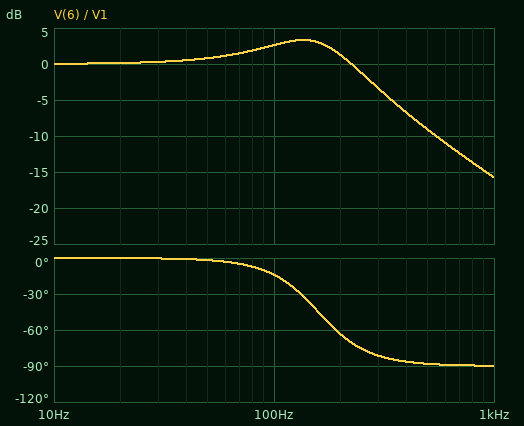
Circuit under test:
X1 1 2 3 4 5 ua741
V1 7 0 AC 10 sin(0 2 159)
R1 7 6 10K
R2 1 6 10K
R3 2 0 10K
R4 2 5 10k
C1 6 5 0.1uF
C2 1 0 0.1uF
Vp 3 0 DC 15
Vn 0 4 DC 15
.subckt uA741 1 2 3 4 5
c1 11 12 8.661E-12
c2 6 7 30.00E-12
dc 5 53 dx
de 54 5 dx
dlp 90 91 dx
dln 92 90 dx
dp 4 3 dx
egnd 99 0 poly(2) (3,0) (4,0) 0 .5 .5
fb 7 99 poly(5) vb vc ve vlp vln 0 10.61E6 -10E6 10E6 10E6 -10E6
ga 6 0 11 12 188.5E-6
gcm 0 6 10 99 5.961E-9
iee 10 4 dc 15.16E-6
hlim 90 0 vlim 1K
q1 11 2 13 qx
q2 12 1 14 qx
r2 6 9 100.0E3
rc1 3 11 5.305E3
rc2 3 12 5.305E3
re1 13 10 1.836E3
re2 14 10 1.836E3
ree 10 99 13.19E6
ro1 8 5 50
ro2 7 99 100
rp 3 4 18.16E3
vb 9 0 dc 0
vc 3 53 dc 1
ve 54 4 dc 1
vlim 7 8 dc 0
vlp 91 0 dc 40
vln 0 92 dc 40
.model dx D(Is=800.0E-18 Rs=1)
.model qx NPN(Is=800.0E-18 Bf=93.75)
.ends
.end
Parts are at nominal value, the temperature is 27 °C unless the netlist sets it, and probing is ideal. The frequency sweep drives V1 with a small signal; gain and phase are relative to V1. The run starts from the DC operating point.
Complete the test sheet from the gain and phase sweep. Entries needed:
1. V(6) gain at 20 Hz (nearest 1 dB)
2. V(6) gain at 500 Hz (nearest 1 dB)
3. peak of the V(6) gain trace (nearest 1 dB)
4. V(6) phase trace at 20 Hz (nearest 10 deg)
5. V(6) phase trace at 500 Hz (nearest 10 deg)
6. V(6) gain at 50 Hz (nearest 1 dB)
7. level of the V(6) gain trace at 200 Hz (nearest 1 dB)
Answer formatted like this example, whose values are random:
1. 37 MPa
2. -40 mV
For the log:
1. 0 dB
2. -9 dB
3. 3 dB
4. 0 deg
5. -90 deg
6. 1 dB
7. 1 dB
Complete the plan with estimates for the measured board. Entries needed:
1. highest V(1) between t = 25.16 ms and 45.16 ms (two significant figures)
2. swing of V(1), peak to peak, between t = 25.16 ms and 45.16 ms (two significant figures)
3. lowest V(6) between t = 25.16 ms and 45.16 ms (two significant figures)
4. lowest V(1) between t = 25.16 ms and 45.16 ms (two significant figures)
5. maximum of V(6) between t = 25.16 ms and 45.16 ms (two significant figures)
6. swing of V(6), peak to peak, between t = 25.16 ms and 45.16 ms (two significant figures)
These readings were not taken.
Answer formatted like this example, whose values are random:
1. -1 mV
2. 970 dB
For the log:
1. 2.0 V
2. 4.0 V
3. -2.8 V
4. -2.0 V
5. 2.8 V
6. 5.7 V
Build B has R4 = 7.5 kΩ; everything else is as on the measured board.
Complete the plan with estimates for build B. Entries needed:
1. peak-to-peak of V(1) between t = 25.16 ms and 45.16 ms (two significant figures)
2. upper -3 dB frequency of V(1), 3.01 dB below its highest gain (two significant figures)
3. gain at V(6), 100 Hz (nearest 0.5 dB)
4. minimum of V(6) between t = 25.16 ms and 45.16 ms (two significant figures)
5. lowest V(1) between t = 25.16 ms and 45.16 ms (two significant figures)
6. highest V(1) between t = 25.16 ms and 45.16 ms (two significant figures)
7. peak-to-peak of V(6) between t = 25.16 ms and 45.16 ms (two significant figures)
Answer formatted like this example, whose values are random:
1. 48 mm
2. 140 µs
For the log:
1. 3.2 V
2. 170 Hz
3. 1.5 dB
4. -2.3 V
5. -1.6 V
6. 1.6 V
7. 4.5 V
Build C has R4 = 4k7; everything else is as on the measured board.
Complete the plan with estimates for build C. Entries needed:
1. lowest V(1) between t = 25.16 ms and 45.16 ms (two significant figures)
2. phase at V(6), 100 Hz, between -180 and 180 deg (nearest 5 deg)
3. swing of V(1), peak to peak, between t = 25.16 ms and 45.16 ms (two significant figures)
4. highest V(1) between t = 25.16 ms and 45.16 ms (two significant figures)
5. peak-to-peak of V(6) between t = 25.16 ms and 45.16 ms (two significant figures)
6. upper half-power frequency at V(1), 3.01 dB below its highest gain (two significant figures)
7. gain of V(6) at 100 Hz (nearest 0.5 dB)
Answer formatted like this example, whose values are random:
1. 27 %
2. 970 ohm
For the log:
1. -1.3 V
2. -25 deg
3. 2.6 V
4. 1.3 V
5. 3.7 V
6. 150 Hz
7. 0.5 dB
